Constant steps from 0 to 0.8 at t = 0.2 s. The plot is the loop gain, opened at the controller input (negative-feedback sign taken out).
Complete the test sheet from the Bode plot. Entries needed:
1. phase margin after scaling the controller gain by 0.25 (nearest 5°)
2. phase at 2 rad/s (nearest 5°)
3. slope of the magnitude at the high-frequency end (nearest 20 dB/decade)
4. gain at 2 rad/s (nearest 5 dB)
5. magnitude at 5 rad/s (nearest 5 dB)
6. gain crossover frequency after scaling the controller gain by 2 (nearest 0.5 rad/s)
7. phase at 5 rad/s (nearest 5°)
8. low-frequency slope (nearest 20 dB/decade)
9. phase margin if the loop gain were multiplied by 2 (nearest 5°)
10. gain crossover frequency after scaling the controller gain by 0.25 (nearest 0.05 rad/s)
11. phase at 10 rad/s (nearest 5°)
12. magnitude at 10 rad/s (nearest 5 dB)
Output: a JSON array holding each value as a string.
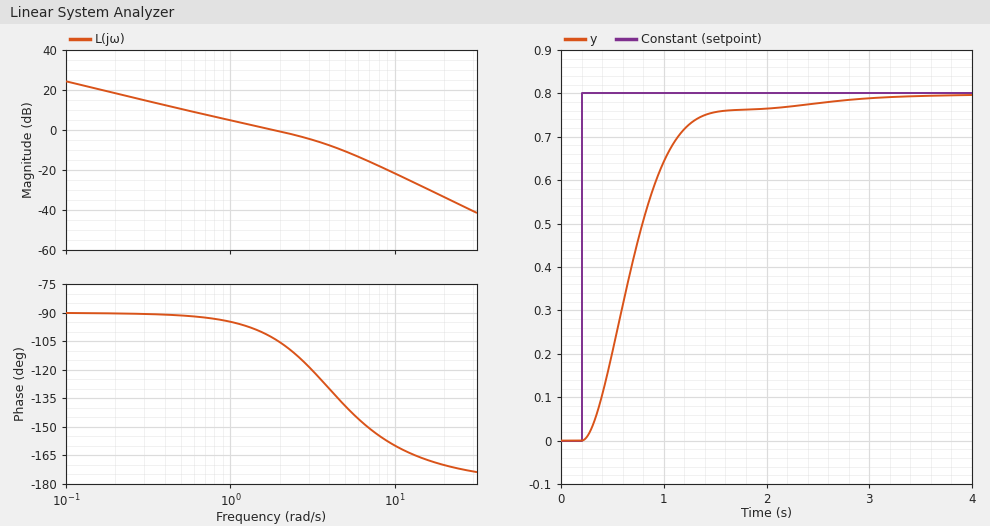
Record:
["90°", "-105°", "-40 dB/decade", "0 dB", "-10 dB", "3.5 rad/s", "-140°", "-20 dB/decade", "55°", "0.40 rad/s", "-160°", "-20 dB"]
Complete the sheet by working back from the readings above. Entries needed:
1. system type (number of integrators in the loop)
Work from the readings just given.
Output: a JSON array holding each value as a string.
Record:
["1"]
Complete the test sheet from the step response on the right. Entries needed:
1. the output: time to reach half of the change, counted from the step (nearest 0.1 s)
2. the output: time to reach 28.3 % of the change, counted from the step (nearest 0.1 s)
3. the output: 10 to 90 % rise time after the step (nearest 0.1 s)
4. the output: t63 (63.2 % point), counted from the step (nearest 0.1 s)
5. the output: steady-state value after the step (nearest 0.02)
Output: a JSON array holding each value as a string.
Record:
["0.5 s", "0.3 s", "0.8 s", "0.6 s", "0.80"]
